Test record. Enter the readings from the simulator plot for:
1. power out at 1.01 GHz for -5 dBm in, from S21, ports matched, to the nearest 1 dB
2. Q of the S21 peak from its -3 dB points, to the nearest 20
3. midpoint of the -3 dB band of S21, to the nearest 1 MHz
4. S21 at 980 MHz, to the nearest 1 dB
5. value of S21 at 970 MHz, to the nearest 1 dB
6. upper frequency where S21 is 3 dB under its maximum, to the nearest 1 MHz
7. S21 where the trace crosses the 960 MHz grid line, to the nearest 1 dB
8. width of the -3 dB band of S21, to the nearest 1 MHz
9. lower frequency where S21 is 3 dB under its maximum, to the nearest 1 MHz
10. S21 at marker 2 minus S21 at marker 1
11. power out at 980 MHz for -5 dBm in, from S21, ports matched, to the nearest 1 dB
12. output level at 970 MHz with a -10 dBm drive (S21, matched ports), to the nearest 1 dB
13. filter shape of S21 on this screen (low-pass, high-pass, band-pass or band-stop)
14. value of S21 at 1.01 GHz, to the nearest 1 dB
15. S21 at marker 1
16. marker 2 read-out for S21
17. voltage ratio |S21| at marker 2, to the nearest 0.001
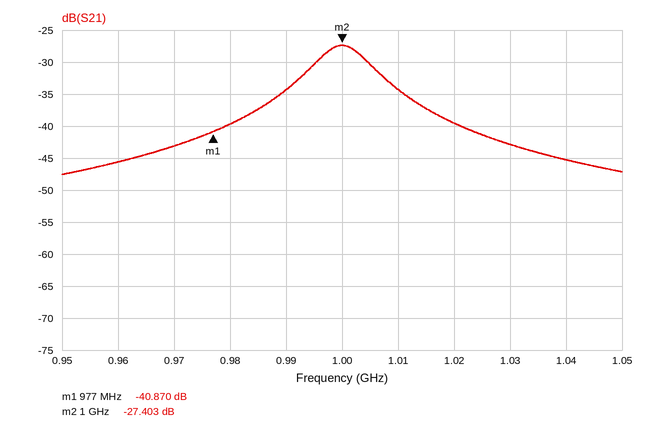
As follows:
-39 dBm
100
1.000 GHz
-40 dB
-43 dB
1.005 GHz
-46 dB
10 MHz
995 MHz
13.467 dB
-45 dBm
-53 dBm
band-pass
-34 dB
-40.870 dB
-27.403 dB
0.043
